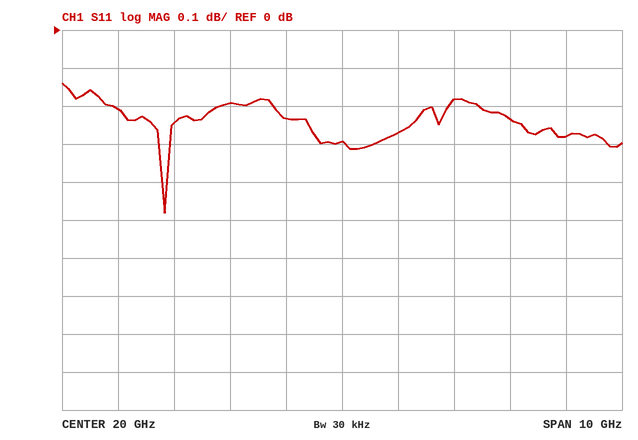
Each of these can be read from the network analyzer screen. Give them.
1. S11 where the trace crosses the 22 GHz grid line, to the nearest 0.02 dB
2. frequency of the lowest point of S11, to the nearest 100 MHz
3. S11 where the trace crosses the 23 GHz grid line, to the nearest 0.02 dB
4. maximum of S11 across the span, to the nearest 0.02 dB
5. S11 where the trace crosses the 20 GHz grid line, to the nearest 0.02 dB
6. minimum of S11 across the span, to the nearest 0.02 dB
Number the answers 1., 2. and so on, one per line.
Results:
1. -0.18 dB
2. 16.8 GHz
3. -0.24 dB
4. -0.14 dB
5. -0.30 dB
6. -0.48 dB
